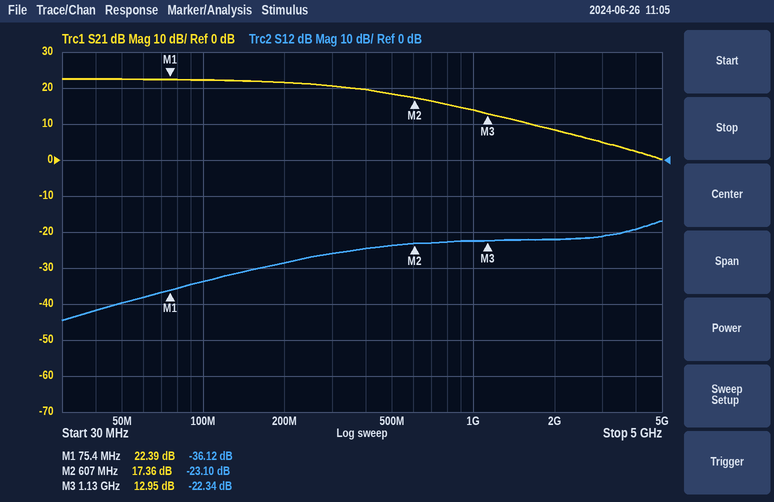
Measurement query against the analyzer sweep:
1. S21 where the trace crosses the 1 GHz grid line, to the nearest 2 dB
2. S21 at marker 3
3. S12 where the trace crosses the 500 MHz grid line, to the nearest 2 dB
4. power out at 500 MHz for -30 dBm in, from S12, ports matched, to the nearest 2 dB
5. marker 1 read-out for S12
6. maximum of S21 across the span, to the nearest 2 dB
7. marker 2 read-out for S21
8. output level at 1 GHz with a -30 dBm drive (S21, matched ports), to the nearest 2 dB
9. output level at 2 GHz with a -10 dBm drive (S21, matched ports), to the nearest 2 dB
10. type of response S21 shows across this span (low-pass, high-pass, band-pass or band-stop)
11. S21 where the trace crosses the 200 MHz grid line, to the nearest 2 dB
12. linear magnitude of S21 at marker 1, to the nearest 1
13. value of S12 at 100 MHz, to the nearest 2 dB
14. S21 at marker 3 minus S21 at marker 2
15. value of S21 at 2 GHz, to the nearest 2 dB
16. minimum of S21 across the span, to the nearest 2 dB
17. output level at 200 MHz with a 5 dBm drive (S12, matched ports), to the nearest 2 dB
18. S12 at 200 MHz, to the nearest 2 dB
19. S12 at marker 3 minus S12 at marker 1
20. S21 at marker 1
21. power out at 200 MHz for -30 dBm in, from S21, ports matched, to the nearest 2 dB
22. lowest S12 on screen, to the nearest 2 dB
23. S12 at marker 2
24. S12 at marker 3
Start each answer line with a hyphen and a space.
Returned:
- 14 dB
- 12.95 dB
- -24 dB
- -54 dBm
- -36.12 dB
- 22 dB
- 17.36 dB
- -16 dBm
- -2 dBm
- low-pass
- 22 dB
- 13
- -34 dB
- -4.41 dB
- 8 dB
- 0 dB
- -24 dBm
- -28 dB
- 13.78 dB
- 22.39 dB
- -8 dBm
- -44 dB
- -23.10 dB
- -22.34 dB
